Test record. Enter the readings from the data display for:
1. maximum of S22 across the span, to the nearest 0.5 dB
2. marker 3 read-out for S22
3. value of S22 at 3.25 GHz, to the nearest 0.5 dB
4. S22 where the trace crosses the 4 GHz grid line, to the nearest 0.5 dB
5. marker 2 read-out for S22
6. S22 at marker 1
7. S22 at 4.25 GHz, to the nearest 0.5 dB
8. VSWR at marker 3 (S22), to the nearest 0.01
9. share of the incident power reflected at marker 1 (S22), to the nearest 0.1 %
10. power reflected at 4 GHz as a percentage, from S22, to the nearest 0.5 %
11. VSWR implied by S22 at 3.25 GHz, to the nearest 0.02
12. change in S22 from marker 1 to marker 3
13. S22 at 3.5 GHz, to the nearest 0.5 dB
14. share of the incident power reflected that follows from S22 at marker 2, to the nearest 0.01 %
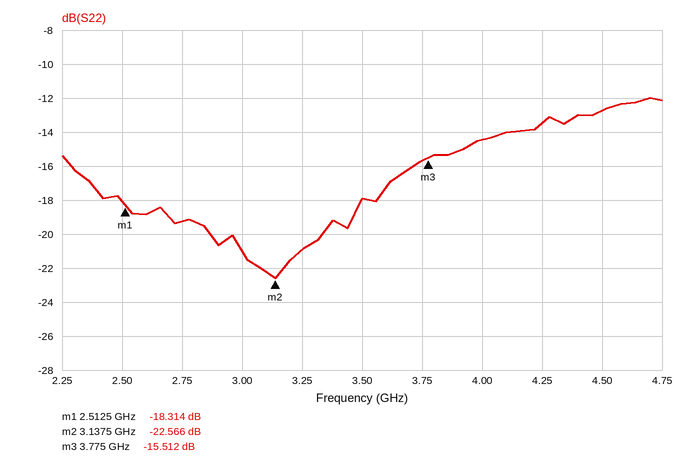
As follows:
-12.0 dB
-15.512 dB
-21.0 dB
-14.5 dB
-22.566 dB
-18.314 dB
-13.5 dB
1.40
1.5 %
3.5 %
1.20
2.802 dB
-18.0 dB
0.55 %
